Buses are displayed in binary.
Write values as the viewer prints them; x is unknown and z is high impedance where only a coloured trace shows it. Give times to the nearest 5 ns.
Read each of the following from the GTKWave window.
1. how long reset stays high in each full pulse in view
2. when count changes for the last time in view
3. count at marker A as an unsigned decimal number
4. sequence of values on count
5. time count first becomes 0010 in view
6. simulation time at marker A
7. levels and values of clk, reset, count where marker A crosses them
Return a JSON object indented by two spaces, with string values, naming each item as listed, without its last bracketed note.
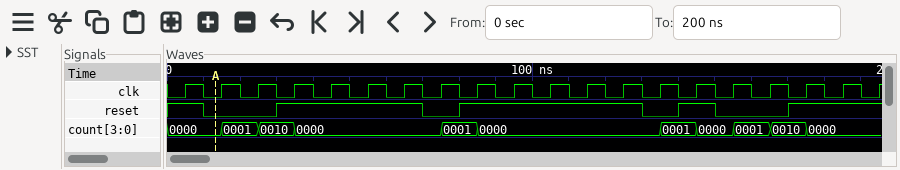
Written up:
{
  "how long reset stays high in each full pulse in view": "40 ns, 50 ns, 10 ns",
  "when count changes for the last time in view": "175 ns",
  "count at marker A as an unsigned decimal number": "0",
  "sequence of values on count": "0000, 0001, 0010, 0000, 0001, 0000, 0001, 0000, 0001, 0010, 0000",
  "time count first becomes 0010 in view": "25 ns",
  "simulation time at marker A": "15 ns",
  "levels and values of clk, reset, count where marker A crosses them": "clk=0, reset=0, count=0000"
}
